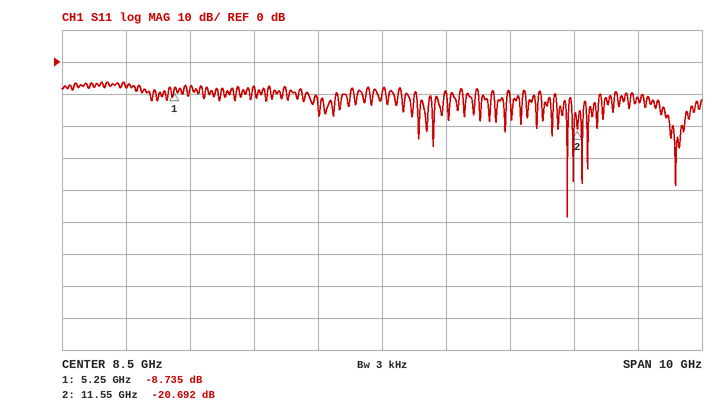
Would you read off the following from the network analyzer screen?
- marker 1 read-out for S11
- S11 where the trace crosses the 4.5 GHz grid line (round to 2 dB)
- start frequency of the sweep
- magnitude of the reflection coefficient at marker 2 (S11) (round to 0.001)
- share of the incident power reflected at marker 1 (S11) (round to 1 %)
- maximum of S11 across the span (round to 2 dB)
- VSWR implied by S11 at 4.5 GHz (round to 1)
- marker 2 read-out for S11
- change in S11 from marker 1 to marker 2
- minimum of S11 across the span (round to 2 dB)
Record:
-8.735 dB
-8 dB
3.5 GHz
0.092
13 %
-6 dB
2
-20.692 dB
-11.957 dB
-48 dB
